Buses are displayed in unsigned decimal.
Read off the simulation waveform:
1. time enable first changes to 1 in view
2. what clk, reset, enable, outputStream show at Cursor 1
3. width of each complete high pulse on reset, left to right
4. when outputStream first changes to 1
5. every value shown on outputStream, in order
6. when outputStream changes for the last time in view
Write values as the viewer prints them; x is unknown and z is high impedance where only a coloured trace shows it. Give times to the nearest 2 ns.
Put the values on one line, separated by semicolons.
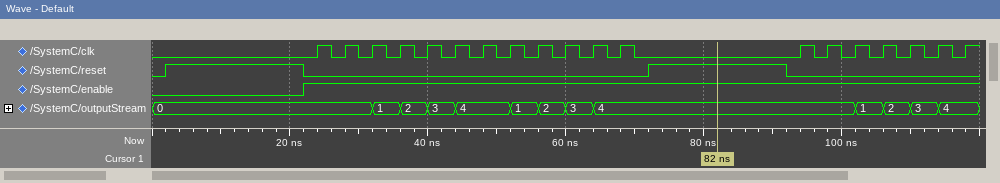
22 ns; clk=0, reset=1, enable=1, outputStream=4; 20 ns, 20 ns; 32 ns; 0, 1, 2, 3, 4, 1, 2, 3, 4, 1, 2, 3, 4; 114 ns
